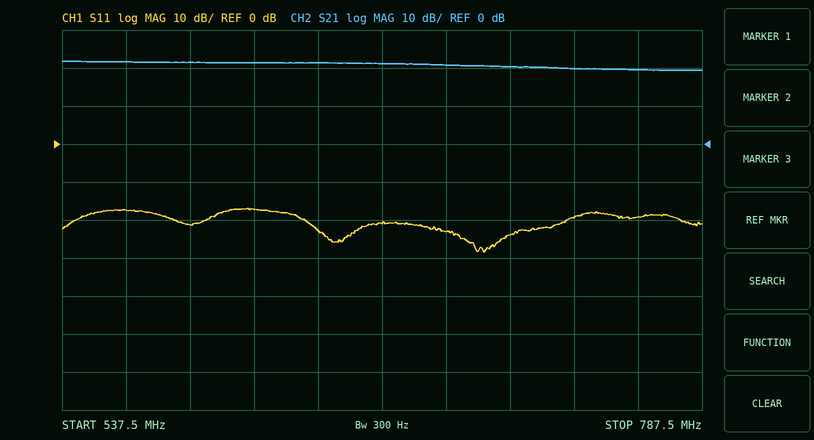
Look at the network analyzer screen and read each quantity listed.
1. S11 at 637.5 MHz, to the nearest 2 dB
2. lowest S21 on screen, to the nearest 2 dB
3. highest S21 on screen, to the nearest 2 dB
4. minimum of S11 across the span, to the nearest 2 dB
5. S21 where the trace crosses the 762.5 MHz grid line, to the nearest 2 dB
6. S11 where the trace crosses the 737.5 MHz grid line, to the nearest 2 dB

-22 dB
20 dB
22 dB
-28 dB
20 dB
-20 dB
